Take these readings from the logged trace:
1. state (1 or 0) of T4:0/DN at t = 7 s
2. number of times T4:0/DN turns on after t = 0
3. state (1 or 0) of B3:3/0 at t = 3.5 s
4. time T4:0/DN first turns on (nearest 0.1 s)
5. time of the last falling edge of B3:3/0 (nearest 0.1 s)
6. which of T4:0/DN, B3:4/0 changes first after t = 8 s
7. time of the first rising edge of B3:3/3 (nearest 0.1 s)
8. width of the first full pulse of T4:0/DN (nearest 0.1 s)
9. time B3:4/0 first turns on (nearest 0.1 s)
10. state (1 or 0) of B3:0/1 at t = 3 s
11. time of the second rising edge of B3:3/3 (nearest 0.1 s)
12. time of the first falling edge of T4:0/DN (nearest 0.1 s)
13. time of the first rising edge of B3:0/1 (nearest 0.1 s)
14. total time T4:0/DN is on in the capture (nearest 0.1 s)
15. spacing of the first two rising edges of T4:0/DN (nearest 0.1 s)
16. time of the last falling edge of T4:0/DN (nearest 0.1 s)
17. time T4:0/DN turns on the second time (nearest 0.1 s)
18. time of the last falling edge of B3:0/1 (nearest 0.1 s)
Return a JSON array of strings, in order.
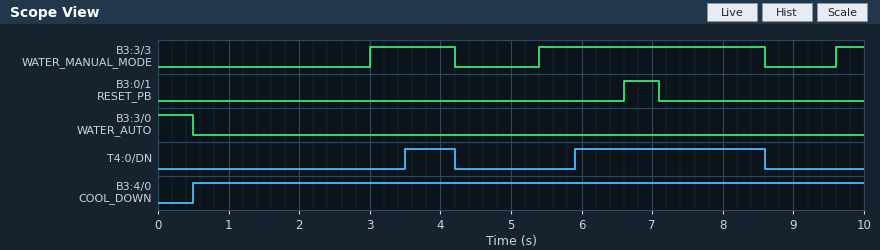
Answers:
["1", "2", "0", "3.5 s", "0.5 s", "T4:0/DN", "3.0 s", "0.7 s", "0.5 s", "0", "5.4 s", "4.2 s", "6.6 s", "3.4 s", "2.4 s", "8.6 s", "5.9 s", "7.1 s"]
